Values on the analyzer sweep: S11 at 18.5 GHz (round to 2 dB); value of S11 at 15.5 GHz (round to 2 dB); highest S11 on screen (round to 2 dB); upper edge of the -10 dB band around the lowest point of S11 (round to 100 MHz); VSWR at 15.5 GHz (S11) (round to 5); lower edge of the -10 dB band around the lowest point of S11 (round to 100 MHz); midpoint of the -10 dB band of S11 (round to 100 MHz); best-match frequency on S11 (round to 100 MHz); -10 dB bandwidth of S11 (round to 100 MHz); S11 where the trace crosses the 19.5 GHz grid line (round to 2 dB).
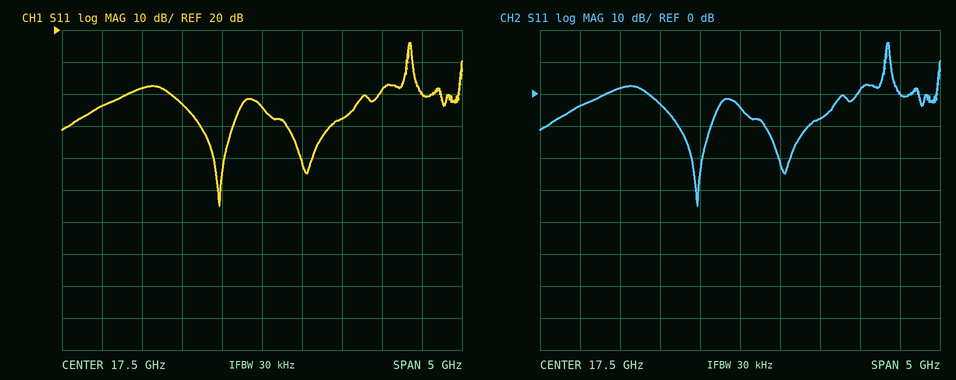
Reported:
-8 dB
-4 dB
16 dB
17.1 GHz
5
16.7 GHz
16.9 GHz
17.0 GHz
400 MHz
0 dB
